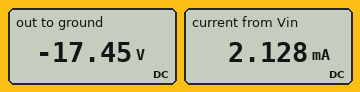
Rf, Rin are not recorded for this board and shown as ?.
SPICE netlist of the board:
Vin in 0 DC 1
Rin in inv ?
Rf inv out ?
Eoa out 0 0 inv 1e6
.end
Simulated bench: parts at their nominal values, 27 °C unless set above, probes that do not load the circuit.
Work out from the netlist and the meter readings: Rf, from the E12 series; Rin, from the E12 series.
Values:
8.2 kΩ
470 Ω
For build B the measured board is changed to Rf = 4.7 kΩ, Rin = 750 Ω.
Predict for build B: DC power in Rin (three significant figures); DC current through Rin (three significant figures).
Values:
1.33 mW
1.33 mA
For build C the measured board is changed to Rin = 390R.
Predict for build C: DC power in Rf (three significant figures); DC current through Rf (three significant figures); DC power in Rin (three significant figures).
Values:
53.9 mW
2.56 mA
2.56 mW
